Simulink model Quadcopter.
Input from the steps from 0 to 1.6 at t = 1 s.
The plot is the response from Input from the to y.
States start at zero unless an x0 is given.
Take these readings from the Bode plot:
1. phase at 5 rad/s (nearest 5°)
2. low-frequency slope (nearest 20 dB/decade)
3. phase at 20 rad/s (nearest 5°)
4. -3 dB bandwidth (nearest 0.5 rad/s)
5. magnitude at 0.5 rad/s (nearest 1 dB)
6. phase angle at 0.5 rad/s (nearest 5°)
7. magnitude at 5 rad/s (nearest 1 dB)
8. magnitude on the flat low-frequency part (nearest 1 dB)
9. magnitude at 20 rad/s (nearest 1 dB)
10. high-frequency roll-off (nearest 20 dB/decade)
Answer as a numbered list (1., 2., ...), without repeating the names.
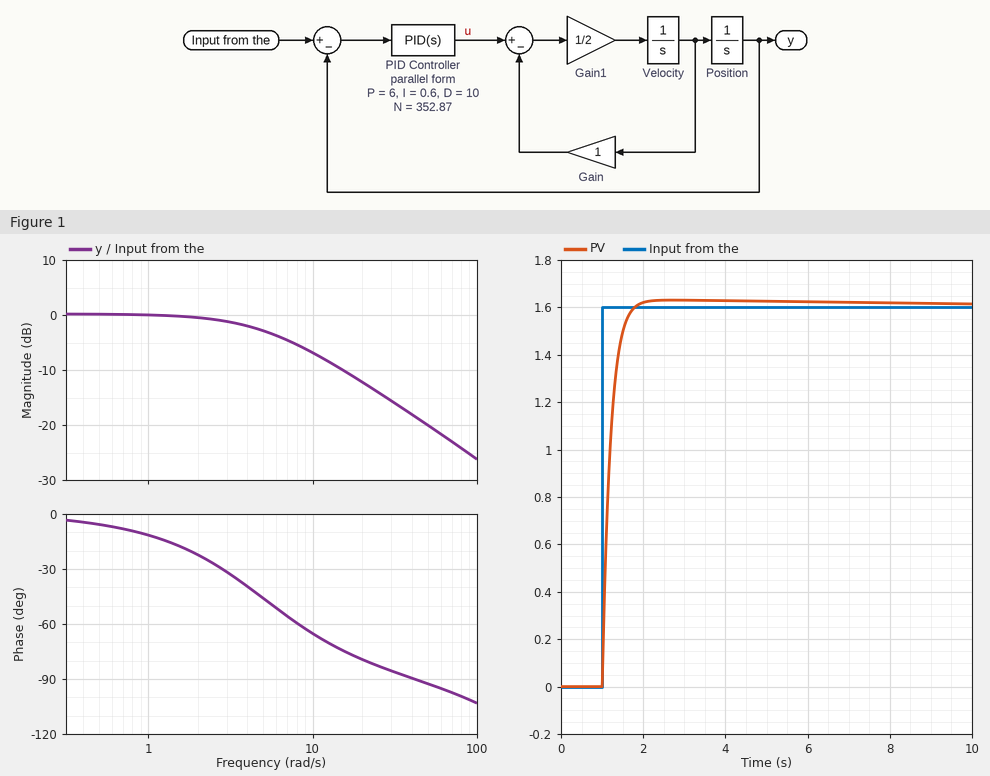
1. -45°
2. 0 dB/decade
3. -80°
4. 5.0 rad/s
5. 0 dB
6. -5°
7. -3 dB
8. 0 dB
9. -12 dB
10. -20 dB/decade
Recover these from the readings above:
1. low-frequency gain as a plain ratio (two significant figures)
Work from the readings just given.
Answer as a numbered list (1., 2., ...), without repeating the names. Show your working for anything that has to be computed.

1. 10^(0 / 20) = 1.0
